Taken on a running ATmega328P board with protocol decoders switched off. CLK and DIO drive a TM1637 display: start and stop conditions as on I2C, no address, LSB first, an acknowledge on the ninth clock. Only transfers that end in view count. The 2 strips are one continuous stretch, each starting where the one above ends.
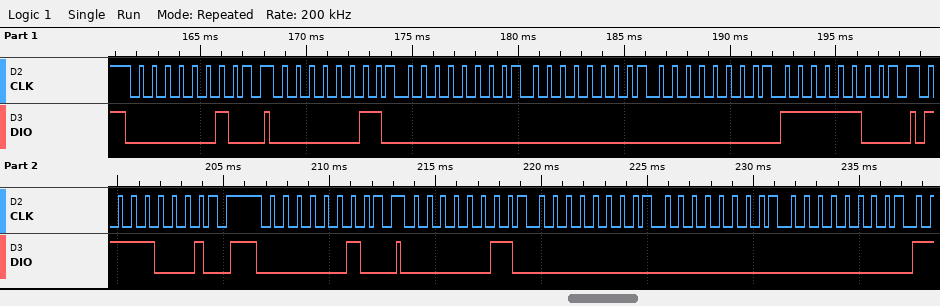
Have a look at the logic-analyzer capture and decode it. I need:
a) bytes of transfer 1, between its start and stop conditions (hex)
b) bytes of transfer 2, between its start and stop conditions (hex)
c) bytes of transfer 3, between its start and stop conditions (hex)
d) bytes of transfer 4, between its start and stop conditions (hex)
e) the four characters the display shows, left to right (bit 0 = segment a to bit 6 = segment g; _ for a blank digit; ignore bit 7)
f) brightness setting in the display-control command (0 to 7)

40
C0 00 00 00 3F
8F
40
___0
7
